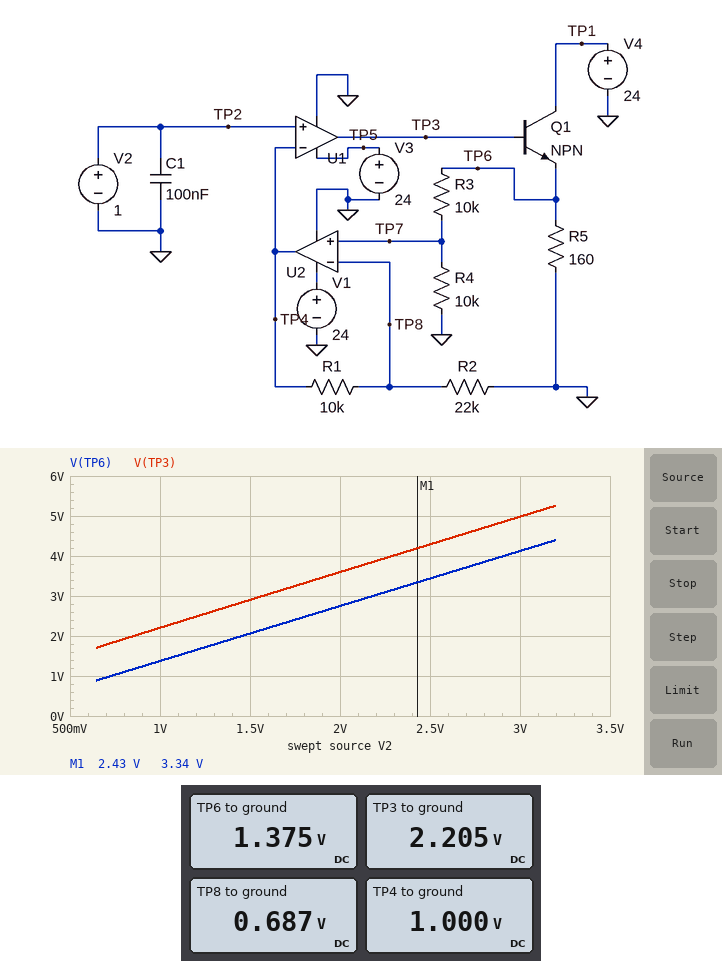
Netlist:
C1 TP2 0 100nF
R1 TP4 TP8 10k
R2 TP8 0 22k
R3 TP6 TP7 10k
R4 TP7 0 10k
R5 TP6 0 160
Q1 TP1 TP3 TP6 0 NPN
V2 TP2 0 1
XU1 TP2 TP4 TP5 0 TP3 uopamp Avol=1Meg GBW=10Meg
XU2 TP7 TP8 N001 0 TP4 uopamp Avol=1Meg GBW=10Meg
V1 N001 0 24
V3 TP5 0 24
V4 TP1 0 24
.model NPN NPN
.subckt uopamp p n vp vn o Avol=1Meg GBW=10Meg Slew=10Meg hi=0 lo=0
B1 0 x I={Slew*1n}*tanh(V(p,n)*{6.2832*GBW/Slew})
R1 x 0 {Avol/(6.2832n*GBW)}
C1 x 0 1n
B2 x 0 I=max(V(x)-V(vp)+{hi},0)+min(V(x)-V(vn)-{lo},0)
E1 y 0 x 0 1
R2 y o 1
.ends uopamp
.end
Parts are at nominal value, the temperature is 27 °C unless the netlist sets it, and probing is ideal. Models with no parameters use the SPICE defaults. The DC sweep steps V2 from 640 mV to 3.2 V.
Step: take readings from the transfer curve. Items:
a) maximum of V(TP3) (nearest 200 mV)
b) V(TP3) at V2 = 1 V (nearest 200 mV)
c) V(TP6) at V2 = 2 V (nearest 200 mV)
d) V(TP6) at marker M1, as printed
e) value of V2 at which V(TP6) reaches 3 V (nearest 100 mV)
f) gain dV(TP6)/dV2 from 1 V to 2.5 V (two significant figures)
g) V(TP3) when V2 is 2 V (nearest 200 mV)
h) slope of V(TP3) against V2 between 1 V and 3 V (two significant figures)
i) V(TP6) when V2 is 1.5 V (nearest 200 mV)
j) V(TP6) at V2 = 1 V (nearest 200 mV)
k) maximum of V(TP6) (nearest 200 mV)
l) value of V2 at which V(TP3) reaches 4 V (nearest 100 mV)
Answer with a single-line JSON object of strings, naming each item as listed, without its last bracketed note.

{"maximum of V(TP3)": "5.2 V", "V(TP3) at V2 = 1 V": "2.2 V", "V(TP6) at V2 = 2 V": "2.8 V", "V(TP6) at marker M1, as printed": "3.34 V", "value of V2 at which V(TP6) reaches 3 V": "2.2 V", "gain dV(TP6)/dV2 from 1 V to 2.5 V": "1.4 V/V", "V(TP3) when V2 is 2 V": "3.6 V", "slope of V(TP3) against V2 between 1 V and 3 V": "1.4 V/V", "V(TP6) when V2 is 1.5 V": "2.0 V", "V(TP6) at V2 = 1 V": "1.4 V", "maximum of V(TP6)": "4.4 V", "value of V2 at which V(TP3) reaches 4 V": "2.3 V"}
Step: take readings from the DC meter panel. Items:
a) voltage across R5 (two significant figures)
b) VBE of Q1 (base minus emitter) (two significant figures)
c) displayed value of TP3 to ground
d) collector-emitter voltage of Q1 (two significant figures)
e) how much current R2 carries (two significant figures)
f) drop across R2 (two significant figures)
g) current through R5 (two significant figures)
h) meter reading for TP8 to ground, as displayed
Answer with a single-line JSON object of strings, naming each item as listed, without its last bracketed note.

{"voltage across R5": "1.4 V", "VBE of Q1 (base minus emitter)": "830 mV", "displayed value of TP3 to ground": "2.205 V", "collector-emitter voltage of Q1": "23 V", "how much current R2 carries": "31 µA", "drop across R2": "690 mV", "current through R5": "8.6 mA", "meter reading for TP8 to ground, as displayed": "0.687 V"}
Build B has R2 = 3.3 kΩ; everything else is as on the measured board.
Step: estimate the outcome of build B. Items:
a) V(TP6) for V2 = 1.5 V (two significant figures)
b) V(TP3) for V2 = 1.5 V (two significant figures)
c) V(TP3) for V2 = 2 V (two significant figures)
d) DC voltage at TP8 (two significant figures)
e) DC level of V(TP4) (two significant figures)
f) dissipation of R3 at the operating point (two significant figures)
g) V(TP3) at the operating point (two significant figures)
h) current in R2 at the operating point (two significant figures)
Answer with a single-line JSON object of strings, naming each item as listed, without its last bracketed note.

{"V(TP6) for V2 = 1.5 V": "740 mV", "V(TP3) for V2 = 1.5 V": "1.6 V", "V(TP3) for V2 = 2 V": "1.8 V", "DC voltage at TP8": "250 mV", "DC level of V(TP4)": "1.0 V", "dissipation of R3 at the operating point": "6.2 µW", "V(TP3) at the operating point": "1.3 V", "current in R2 at the operating point": "75 µA"}
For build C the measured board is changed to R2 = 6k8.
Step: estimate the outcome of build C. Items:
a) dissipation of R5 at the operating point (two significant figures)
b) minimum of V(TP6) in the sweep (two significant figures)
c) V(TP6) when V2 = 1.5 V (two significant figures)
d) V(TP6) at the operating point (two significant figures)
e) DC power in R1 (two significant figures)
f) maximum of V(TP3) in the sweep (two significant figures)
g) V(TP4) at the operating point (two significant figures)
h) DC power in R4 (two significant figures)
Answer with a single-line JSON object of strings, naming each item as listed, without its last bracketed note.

{"dissipation of R5 at the operating point": "4.1 mW", "minimum of V(TP6) in the sweep": "520 mV", "V(TP6) when V2 = 1.5 V": "1.2 V", "V(TP6) at the operating point": "810 mV", "DC power in R1": "35 µW", "maximum of V(TP3) in the sweep": "3.4 V", "V(TP4) at the operating point": "1.0 V", "DC power in R4": "16 µW"}
